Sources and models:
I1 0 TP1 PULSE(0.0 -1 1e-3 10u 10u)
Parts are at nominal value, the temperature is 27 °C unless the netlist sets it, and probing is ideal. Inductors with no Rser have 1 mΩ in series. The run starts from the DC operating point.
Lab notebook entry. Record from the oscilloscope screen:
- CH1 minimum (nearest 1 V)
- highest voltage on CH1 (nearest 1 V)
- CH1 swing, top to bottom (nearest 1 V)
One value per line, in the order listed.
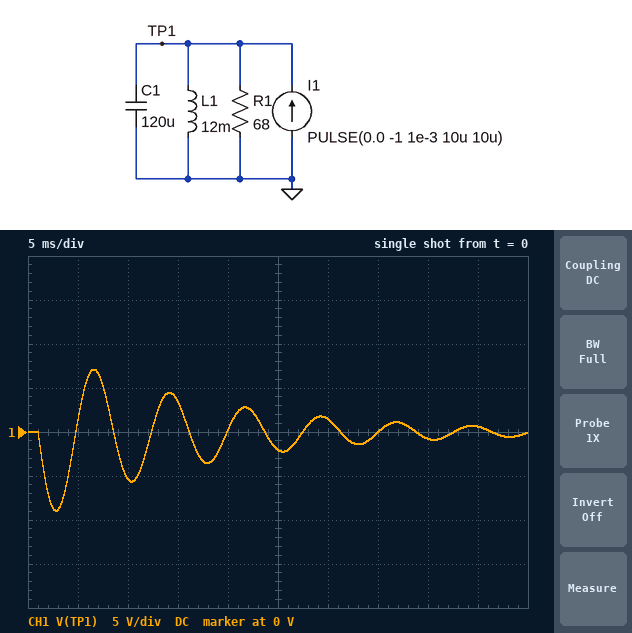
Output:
-9 V
7 V
16 V
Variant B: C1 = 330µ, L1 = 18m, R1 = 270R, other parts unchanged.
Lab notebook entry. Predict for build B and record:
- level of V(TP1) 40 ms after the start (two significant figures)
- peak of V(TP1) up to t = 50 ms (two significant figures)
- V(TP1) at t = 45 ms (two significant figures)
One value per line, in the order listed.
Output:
1.7 V
6.9 V
4.1 V
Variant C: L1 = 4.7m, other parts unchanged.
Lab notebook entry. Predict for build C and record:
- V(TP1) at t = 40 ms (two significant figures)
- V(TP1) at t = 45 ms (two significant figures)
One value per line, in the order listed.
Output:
-570 mV
-390 mV
